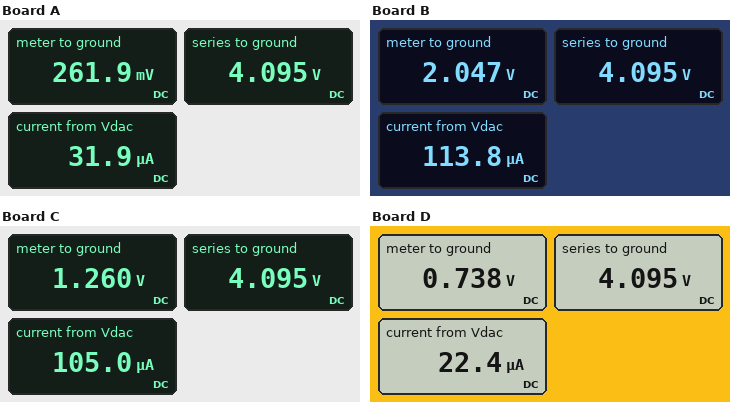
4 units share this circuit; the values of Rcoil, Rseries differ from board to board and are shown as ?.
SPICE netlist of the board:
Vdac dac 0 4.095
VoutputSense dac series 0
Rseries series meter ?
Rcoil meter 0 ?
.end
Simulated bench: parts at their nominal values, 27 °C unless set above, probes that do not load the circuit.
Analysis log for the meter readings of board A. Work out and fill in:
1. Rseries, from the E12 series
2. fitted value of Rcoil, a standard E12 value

120 kΩ
8.2 kΩ
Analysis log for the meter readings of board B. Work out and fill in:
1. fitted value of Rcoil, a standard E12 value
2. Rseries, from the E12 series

18 kΩ
18 kΩ
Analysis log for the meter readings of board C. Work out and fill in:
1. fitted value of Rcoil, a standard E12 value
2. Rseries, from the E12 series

12 kΩ
27 kΩ
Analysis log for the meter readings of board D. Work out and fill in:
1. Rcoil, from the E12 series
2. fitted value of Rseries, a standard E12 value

33 kΩ
150 kΩ
